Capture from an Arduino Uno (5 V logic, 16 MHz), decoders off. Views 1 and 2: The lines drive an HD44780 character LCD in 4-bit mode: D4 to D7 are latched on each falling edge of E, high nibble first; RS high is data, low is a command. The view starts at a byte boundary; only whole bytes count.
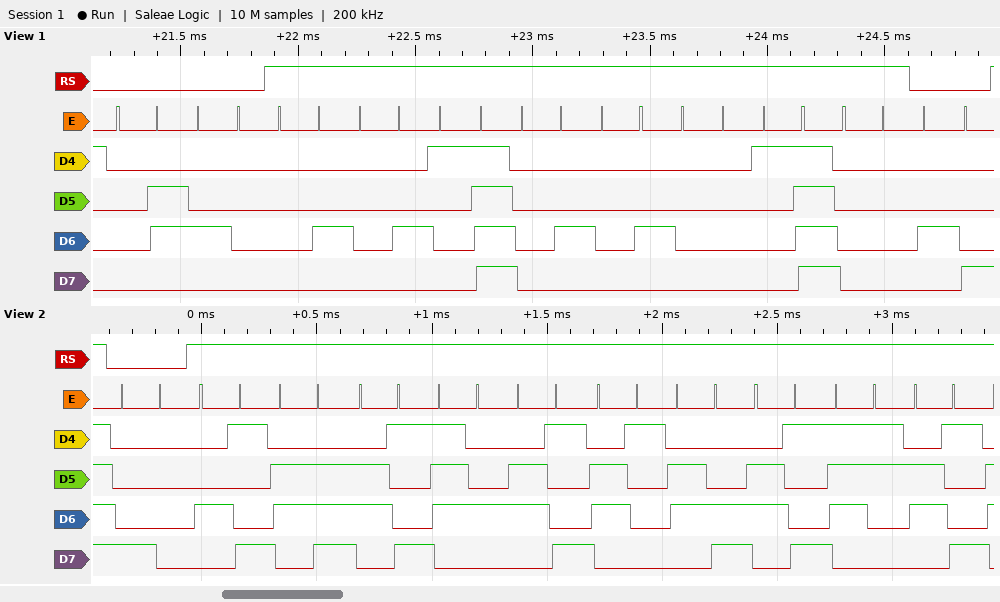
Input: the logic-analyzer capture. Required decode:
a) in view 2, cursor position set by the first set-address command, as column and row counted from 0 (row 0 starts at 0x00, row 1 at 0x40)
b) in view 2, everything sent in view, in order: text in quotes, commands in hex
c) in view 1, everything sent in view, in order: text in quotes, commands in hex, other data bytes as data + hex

column 0, row 0
0x80 "Initialisi"
0x06 0x40 data 04 04 1F 04 04 00 1F 00 0x48
